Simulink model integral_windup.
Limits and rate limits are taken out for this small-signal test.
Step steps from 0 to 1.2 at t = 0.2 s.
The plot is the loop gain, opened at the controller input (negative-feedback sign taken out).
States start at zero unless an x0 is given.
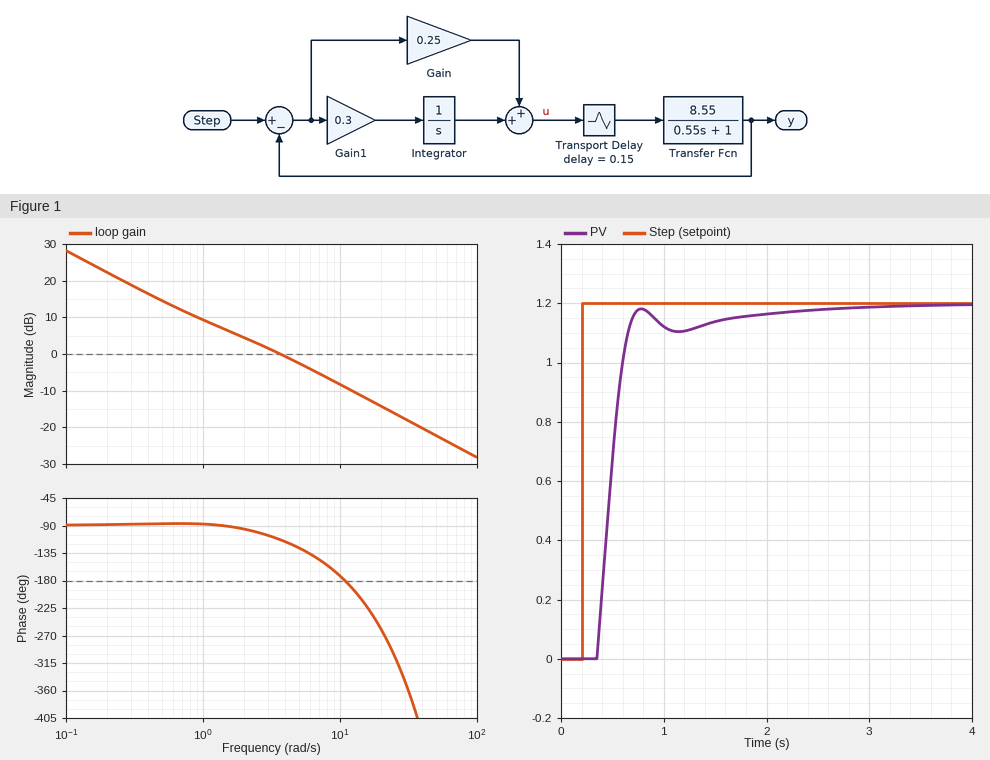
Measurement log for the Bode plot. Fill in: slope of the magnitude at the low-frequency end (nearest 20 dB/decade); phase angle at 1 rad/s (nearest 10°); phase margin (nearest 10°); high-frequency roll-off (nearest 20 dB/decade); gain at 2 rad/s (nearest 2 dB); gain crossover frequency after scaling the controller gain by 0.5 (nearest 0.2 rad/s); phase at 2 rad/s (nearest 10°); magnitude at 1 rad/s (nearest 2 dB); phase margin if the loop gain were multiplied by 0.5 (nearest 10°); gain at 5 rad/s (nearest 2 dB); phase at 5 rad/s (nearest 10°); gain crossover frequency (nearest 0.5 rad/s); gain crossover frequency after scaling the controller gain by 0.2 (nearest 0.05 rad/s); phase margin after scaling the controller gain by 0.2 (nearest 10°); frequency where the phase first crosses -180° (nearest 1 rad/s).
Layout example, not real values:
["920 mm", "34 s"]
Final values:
["-20 dB/decade", "-90°", "70°", "-20 dB/decade", "4 dB", "1.6 rad/s", "-100°", "10 dB", "90°", "-2 dB", "-130°", "3.5 rad/s", "0.55 rad/s", "90°", "11 rad/s"]
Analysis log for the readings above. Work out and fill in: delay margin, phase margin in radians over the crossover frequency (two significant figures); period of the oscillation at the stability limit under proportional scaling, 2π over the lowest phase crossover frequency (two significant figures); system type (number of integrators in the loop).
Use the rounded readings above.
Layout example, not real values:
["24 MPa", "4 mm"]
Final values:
["0.35 s", "0.57 s", "1"]
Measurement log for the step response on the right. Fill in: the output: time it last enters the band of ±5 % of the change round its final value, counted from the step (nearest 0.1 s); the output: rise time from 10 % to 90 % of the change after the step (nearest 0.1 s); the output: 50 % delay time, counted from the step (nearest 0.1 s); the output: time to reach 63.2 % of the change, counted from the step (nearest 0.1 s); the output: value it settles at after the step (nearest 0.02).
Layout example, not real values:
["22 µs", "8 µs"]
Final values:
["1.3 s", "0.3 s", "0.3 s", "0.3 s", "1.20"]
